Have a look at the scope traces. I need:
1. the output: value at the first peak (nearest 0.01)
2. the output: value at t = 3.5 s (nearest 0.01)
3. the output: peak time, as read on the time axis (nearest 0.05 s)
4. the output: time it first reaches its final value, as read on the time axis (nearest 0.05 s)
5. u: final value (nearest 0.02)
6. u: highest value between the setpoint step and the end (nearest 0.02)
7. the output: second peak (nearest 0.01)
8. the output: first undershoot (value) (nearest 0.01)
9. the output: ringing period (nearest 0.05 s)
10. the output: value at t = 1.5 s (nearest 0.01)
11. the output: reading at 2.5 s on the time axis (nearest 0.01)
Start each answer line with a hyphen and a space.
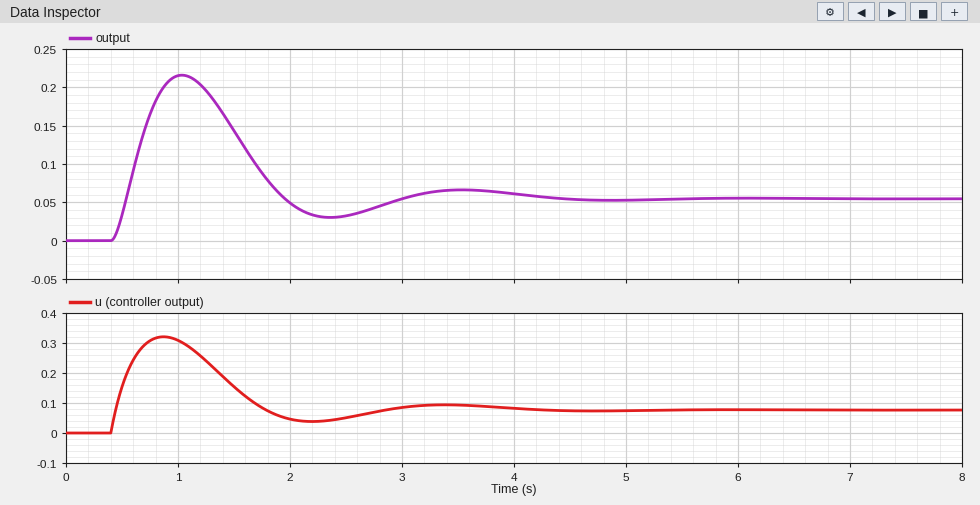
- 0.22
- 0.07
- 1.05 s
- 0.55 s
- 0.08
- 0.32
- 0.07
- 0.03
- 2.50 s
- 0.14
- 0.03
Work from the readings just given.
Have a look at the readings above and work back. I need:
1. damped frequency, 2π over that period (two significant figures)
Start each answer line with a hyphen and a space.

- 2.5 rad/s
